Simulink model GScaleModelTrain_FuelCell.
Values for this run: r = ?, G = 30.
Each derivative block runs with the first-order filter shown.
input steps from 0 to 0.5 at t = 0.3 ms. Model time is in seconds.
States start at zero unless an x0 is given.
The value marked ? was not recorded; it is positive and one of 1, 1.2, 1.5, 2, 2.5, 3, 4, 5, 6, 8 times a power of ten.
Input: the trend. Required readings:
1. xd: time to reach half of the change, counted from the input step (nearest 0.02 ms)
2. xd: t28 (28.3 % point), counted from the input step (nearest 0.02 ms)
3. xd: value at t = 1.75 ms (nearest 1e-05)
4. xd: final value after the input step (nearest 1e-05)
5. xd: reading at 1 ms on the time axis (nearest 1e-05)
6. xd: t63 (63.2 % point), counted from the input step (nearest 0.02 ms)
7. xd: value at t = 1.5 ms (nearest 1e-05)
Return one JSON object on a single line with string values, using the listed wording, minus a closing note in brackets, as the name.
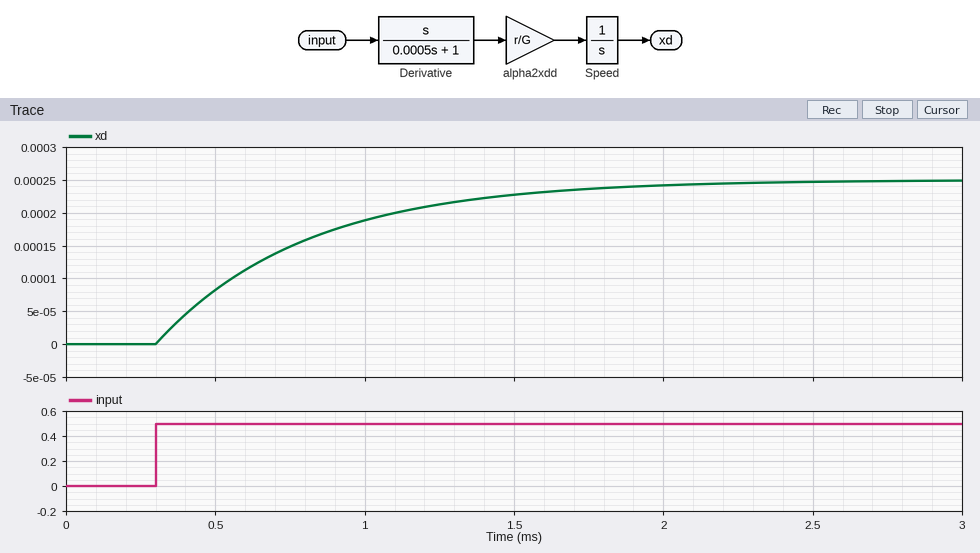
{"xd: time to reach half of the change, counted from the input step": "0.34 ms", "xd: t28 (28.3 % point), counted from the input step": "0.16 ms", "xd: value at t = 1.75 ms": "0.00024", "xd: final value after the input step": "0.00025", "xd: reading at 1 ms on the time axis": "0.00019", "xd: t63 (63.2 % point), counted from the input step": "0.50 ms", "xd: value at t = 1.5 ms": "0.00023"}
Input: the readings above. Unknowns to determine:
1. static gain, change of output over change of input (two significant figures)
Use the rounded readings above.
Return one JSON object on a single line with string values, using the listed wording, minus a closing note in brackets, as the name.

{"static gain, change of output over change of input": "0.00050"}
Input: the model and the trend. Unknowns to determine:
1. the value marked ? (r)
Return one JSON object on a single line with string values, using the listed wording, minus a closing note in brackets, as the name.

{"the value marked ?": "0.015"}
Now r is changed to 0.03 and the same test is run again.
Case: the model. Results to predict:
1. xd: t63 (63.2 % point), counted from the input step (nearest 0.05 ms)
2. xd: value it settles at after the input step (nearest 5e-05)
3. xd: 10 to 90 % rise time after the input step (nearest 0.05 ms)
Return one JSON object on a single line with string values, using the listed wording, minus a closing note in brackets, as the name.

{"xd: t63 (63.2 % point), counted from the input step": "0.50 ms", "xd: value it settles at after the input step": "0.00050", "xd: 10 to 90 % rise time after the input step": "1.10 ms"}
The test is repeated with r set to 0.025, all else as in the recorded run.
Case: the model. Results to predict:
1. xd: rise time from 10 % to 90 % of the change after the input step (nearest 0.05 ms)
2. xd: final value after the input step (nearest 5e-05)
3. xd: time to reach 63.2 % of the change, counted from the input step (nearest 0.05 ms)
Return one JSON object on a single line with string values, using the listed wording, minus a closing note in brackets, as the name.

{"xd: rise time from 10 % to 90 % of the change after the input step": "1.10 ms", "xd: final value after the input step": "0.00040", "xd: time to reach 63.2 % of the change, counted from the input step": "0.50 ms"}
